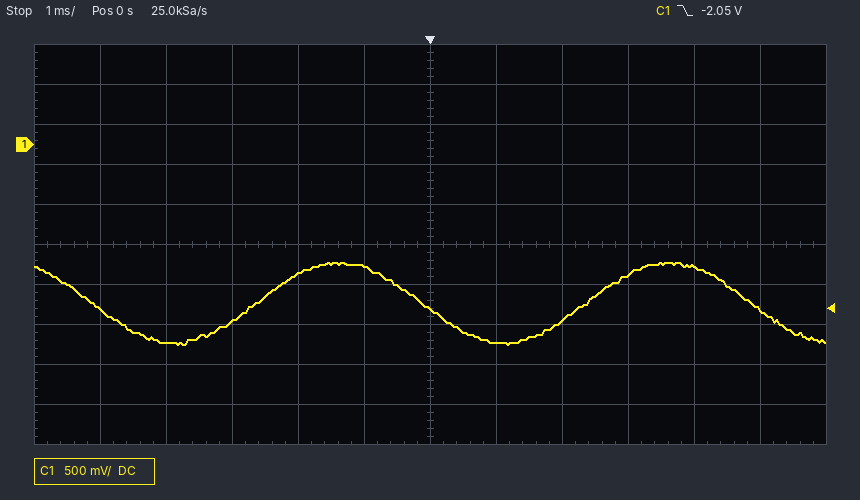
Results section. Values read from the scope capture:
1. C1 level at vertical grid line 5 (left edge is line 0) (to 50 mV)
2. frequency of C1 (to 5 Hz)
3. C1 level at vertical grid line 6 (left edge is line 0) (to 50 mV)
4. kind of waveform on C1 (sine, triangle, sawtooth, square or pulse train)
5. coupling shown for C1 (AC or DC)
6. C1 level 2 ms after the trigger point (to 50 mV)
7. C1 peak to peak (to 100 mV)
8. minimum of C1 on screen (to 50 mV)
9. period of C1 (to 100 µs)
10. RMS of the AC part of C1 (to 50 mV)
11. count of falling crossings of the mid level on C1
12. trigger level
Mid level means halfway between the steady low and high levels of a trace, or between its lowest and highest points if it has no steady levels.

-1.50 V
200 Hz
-2.05 V
sine
DC
-2.20 V
1.00 V
-2.50 V
5.0 ms
350 mV
3
-2.05 V
